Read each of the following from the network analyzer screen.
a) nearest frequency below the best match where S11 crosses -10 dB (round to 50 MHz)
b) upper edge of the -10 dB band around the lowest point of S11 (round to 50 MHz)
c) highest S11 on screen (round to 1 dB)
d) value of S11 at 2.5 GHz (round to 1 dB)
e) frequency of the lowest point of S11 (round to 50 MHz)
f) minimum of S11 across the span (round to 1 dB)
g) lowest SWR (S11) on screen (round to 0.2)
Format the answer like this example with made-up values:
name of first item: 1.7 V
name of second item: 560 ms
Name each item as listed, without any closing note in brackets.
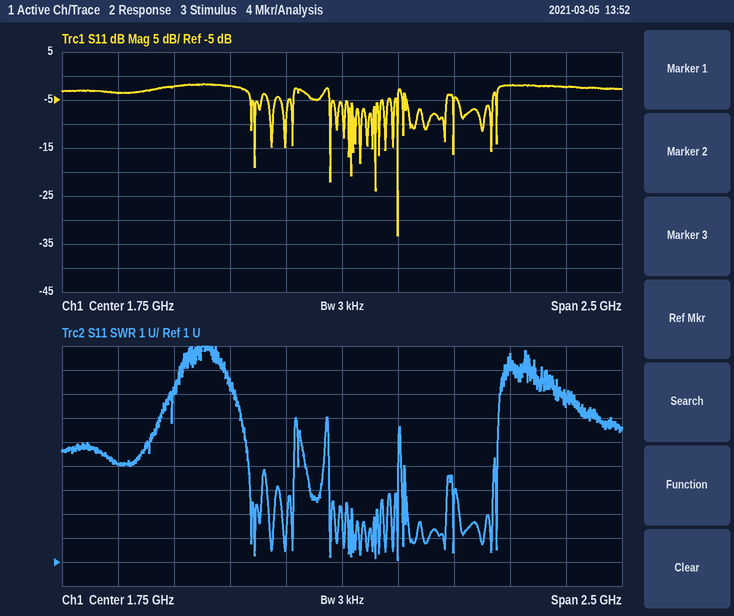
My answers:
nearest frequency below the best match where S11 crosses -10 dB: 2.00 GHz
upper edge of the -10 dB band around the lowest point of S11: 2.00 GHz
highest S11 on screen: -2 dB
value of S11 at 2.5 GHz: -2 dB
frequency of the lowest point of S11: 2.00 GHz
minimum of S11 across the span: -33 dB
lowest SWR (S11) on screen: 1.0
